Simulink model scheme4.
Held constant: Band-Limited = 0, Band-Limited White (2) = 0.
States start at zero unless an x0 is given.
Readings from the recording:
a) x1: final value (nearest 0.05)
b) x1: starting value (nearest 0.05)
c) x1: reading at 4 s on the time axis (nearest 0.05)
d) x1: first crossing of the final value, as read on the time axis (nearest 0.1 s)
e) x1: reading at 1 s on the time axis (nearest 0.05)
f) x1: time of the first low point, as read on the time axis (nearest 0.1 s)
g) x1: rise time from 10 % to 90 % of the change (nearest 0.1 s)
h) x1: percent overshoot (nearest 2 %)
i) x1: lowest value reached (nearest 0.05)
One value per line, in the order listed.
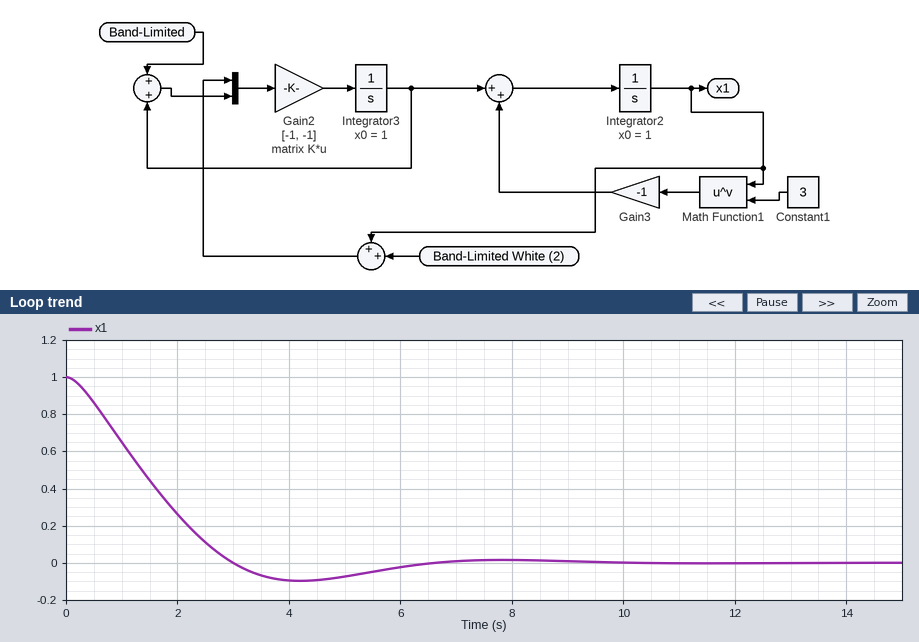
0.00
1.00
-0.10
3.0 s
0.65
4.2 s
2.1 s
10 %
-0.10
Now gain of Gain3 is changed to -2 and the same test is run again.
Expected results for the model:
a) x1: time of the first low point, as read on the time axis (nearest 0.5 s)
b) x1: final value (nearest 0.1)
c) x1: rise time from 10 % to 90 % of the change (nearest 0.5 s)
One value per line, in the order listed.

4.5 s
0.0
2.5 s
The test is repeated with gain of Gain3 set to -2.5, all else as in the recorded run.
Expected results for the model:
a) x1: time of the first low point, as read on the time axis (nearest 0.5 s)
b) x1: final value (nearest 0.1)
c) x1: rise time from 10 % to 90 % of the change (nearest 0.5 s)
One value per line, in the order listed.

4.5 s
0.0
2.5 s
